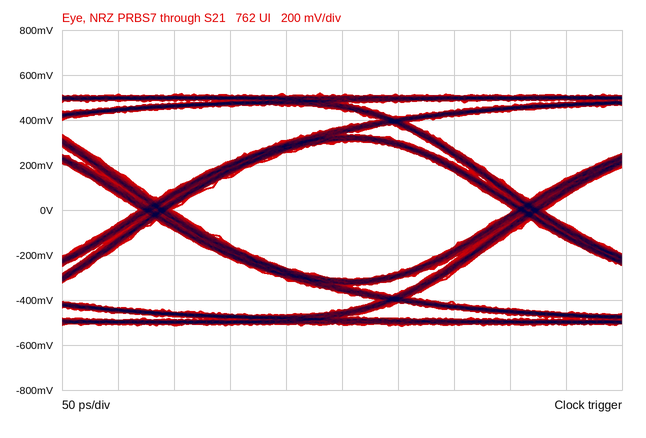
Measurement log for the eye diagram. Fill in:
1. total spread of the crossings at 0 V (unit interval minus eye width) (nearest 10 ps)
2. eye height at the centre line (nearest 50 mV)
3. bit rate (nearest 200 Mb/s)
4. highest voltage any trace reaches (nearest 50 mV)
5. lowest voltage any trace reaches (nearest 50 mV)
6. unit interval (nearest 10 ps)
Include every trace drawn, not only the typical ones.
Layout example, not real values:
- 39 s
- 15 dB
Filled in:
- 30 ps
- 600 mV
- 3.0 Gb/s
- 500 mV
- -500 mV
- 330 ps
